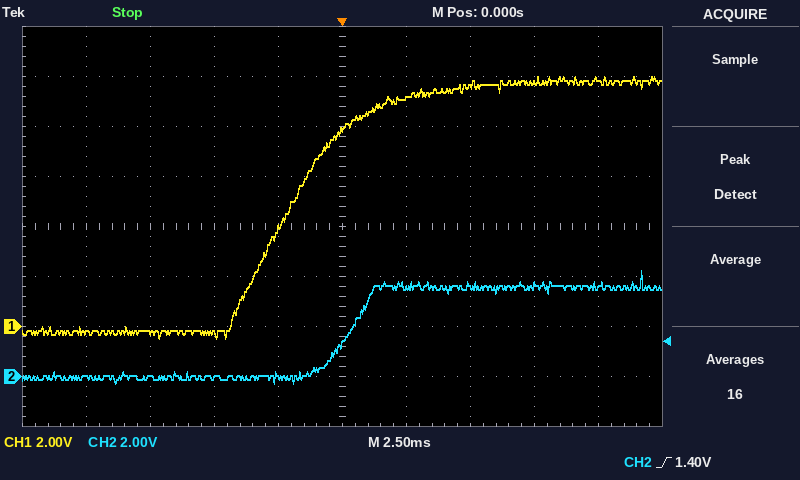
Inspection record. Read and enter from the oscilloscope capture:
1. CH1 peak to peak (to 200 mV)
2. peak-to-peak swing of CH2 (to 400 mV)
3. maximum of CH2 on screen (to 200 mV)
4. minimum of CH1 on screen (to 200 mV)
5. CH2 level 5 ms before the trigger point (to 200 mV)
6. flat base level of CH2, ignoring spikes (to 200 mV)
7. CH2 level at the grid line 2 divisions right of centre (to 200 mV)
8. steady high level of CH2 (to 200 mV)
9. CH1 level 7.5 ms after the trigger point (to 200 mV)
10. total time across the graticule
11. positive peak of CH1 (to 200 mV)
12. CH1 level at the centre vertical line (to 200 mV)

10.4 V
4.4 V
4.2 V
-400 mV
0.0 V
0.0 V
3.6 V
3.6 V
9.8 V
25 ms
10.0 V
7.8 V
